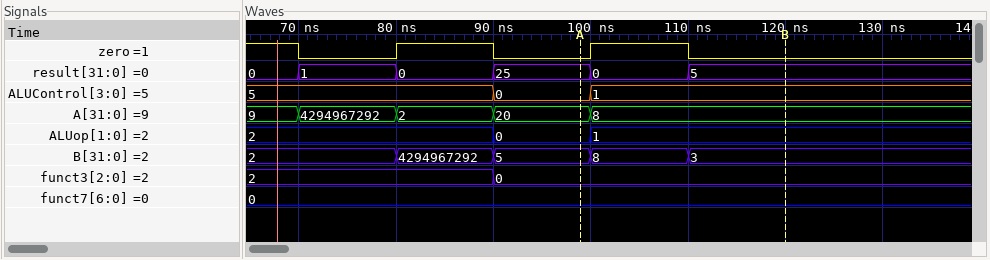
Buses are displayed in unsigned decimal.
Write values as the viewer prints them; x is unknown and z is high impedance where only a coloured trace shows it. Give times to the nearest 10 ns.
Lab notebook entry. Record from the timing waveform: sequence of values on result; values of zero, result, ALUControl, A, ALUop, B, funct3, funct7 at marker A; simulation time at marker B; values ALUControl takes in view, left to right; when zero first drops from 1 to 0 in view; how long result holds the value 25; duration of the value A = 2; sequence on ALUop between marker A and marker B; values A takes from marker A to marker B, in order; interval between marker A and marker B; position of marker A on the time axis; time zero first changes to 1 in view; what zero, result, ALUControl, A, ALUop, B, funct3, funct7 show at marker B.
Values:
0, 1, 0, 25, 0, 5
zero=0, result=25, ALUControl=0, A=20, ALUop=0, B=5, funct3=0, funct7=0
120 ns
5, 0, 1
70 ns
10 ns
10 ns
0, 1
20, 8
20 ns
100 ns
80 ns
zero=0, result=5, ALUControl=1, A=8, ALUop=1, B=3, funct3=0, funct7=0
